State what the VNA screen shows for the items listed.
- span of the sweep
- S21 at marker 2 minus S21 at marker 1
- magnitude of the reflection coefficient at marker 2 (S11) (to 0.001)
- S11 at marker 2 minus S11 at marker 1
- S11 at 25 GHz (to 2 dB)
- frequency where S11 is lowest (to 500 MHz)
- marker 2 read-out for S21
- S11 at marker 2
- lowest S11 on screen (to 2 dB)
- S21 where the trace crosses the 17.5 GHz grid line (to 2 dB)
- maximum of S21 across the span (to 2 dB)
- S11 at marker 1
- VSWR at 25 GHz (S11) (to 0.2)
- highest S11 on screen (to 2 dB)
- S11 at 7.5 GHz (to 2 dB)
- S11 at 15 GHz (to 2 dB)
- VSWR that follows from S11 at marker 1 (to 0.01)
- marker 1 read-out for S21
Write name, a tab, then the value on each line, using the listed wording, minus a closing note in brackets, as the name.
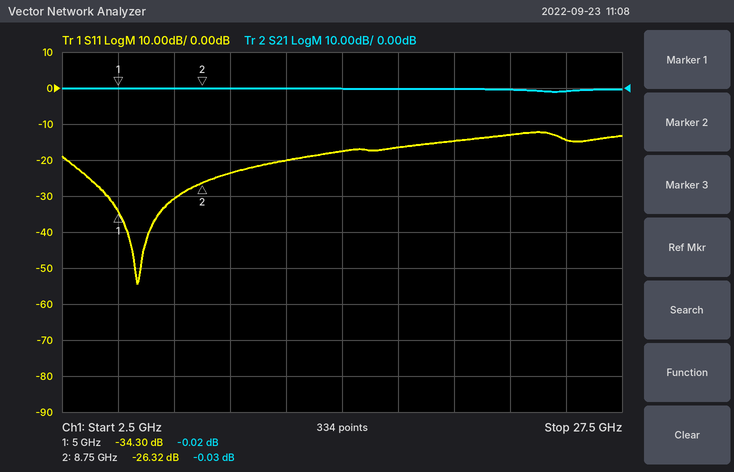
span of the sweep	25 GHz
S21 at marker 2 minus S21 at marker 1	-0.01 dB
magnitude of the reflection coefficient at marker 2 (S11)	0.048
S11 at marker 2 minus S11 at marker 1	7.98 dB
S11 at 25 GHz	-14 dB
frequency where S11 is lowest	6.0 GHz
marker 2 read-out for S21	-0.03 dB
S11 at marker 2	-26.32 dB
lowest S11 on screen	-54 dB
S21 where the trace crosses the 17.5 GHz grid line	0 dB
maximum of S21 across the span	0 dB
S11 at marker 1	-34.30 dB
VSWR at 25 GHz (S11)	1.4
highest S11 on screen	-12 dB
S11 at 7.5 GHz	-30 dB
S11 at 15 GHz	-18 dB
VSWR that follows from S11 at marker 1	1.04
marker 1 read-out for S21	-0.02 dB
